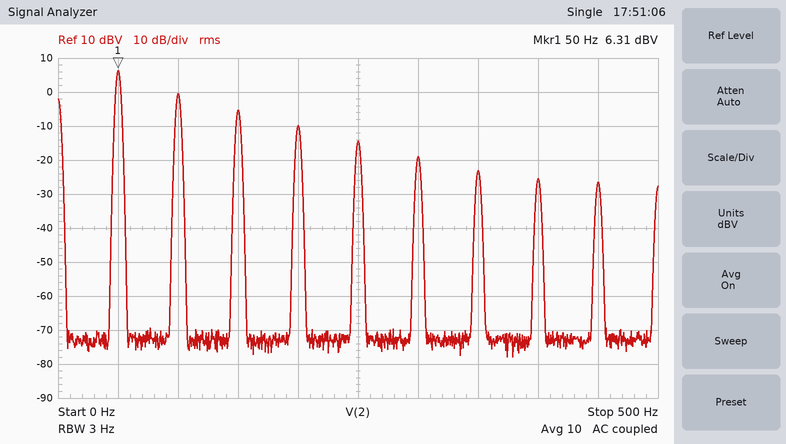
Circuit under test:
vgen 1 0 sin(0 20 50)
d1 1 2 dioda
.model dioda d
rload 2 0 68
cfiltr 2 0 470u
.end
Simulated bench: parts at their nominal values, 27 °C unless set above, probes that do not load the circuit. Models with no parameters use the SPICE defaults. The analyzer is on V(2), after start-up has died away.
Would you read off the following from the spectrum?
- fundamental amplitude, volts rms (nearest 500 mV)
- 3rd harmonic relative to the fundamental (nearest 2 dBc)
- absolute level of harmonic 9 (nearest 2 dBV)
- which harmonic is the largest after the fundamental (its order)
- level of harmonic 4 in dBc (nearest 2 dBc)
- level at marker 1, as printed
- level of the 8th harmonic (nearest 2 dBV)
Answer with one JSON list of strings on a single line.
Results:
["2.0 V", "-12 dBc", "-26 dBV", "2", "-16 dBc", "6.31 dBV", "-26 dBV"]
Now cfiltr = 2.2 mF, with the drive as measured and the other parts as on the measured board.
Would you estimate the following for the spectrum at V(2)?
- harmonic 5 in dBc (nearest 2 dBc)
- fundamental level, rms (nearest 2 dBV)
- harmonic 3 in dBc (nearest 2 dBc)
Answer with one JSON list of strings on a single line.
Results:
["-16 dBc", "-6 dBV", "-10 dBc"]
